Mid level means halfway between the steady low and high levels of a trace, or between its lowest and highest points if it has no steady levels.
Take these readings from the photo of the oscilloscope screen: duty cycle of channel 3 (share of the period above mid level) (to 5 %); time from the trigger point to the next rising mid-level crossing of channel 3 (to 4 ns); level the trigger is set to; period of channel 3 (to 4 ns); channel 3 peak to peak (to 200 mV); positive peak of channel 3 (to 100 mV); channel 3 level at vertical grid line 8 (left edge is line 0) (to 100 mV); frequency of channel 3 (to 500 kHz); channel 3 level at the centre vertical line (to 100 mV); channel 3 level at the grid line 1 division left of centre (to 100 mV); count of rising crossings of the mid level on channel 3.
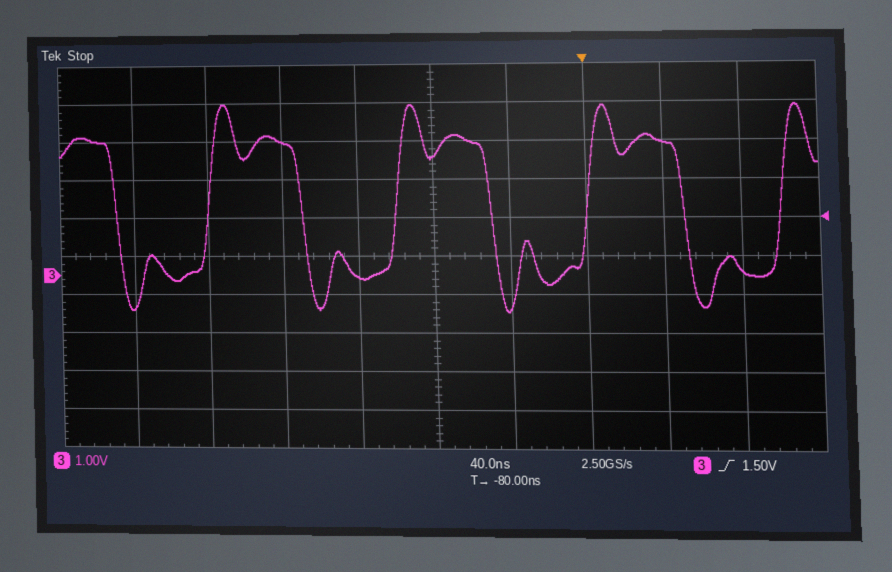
50 %
100 ns
1.50 V
100 ns
5.4 V
4.5 V
3.5 V
10.0 MHz
3.1 V
0.0 V
4
